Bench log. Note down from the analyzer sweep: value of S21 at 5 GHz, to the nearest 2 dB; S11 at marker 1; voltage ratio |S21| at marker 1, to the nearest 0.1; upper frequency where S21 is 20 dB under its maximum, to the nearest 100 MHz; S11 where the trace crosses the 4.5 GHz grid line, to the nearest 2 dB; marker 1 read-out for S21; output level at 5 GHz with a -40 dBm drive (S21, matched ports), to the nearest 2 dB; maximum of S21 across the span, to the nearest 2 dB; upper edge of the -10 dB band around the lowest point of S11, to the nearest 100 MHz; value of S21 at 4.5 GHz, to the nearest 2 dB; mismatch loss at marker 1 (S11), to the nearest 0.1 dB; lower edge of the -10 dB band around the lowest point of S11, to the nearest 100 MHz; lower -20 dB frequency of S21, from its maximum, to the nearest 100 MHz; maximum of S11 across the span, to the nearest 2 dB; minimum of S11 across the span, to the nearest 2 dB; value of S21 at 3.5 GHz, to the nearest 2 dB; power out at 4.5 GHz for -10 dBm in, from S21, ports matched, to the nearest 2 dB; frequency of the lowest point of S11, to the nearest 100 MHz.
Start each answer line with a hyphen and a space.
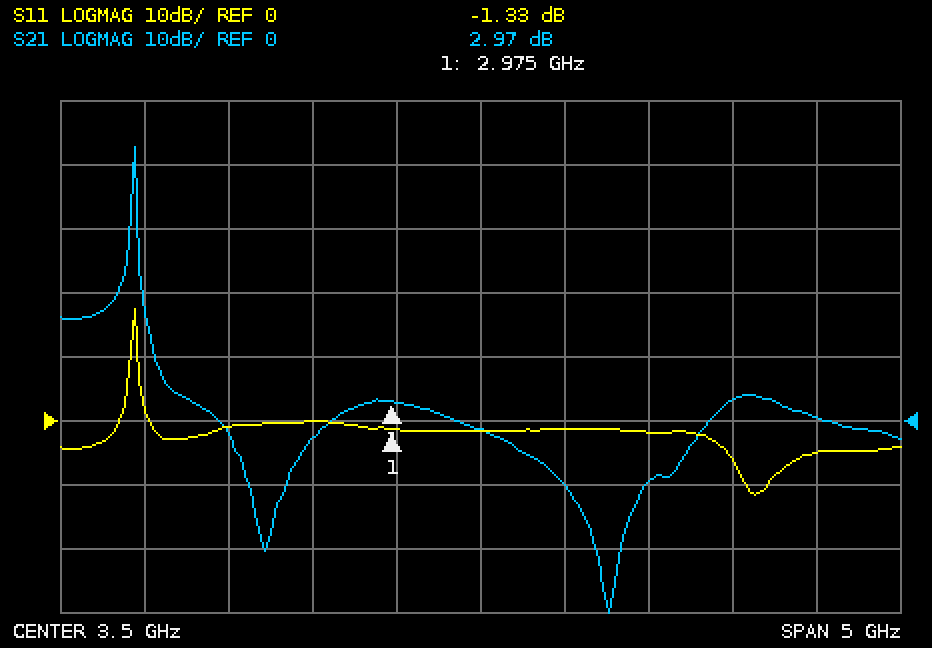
- 4 dB
- -1.33 dB
- 1.4
- 1.5 GHz
- -2 dB
- 2.97 dB
- -36 dBm
- 42 dB
- 5.2 GHz
- -10 dB
- 5.8 dB
- 5.1 GHz
- 1.4 GHz
- 18 dB
- -12 dB
- -2 dB
- -20 dBm
- 5.1 GHz
